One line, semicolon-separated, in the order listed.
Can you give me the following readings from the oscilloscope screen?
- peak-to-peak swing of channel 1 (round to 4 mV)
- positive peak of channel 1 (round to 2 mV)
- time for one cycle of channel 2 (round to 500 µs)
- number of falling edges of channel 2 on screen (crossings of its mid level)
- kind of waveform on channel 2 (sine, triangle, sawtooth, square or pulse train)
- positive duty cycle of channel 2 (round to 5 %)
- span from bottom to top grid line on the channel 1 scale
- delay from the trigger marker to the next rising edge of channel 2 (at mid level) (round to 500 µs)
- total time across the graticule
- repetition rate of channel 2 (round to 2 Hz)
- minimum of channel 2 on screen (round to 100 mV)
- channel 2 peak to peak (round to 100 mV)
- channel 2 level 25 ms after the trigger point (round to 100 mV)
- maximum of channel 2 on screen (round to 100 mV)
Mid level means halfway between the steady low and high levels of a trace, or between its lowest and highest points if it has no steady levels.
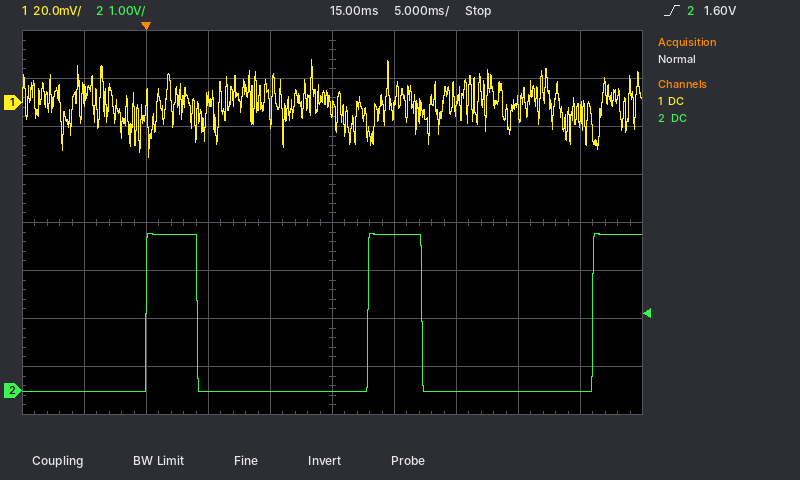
40 mV; 18 mV; 18.0 ms; 2; pulse train; 25 %; 160 mV; 18.0 ms; 50 ms; 56 Hz; 0.0 V; 3.3 V; 0.0 V; 3.3 V
